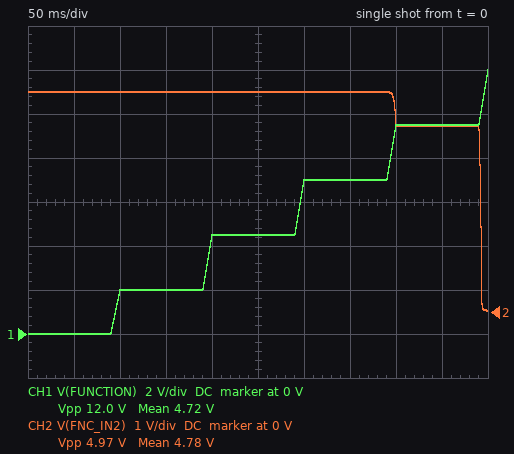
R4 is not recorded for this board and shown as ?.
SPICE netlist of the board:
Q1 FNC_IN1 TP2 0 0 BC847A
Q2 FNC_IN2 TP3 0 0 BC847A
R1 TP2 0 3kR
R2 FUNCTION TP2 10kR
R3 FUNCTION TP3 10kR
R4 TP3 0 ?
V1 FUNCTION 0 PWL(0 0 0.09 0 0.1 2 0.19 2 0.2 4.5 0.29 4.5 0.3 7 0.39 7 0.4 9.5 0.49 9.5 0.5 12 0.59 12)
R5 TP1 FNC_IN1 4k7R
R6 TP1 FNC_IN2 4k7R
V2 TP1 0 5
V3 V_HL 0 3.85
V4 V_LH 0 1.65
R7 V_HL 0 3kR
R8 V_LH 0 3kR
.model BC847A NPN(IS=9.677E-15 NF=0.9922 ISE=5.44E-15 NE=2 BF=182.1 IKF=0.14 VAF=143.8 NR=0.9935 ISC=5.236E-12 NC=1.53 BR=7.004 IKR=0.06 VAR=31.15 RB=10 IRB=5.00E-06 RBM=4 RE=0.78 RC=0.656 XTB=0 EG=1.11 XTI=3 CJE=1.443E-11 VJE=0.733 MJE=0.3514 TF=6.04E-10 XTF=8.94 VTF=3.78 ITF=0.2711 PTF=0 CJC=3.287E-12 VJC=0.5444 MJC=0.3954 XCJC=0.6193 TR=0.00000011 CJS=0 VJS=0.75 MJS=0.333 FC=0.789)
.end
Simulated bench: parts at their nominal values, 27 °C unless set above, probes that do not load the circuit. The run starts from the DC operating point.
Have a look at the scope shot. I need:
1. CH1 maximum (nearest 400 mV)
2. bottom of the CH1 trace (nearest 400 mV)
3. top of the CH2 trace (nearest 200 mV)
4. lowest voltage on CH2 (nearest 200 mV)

12.0 V
0 V
5.0 V
0 V
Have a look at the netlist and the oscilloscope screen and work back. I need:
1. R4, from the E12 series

680 Ω
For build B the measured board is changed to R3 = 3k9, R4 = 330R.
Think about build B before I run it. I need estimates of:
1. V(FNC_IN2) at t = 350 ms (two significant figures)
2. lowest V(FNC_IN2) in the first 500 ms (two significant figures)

4.9 V
12 mV
